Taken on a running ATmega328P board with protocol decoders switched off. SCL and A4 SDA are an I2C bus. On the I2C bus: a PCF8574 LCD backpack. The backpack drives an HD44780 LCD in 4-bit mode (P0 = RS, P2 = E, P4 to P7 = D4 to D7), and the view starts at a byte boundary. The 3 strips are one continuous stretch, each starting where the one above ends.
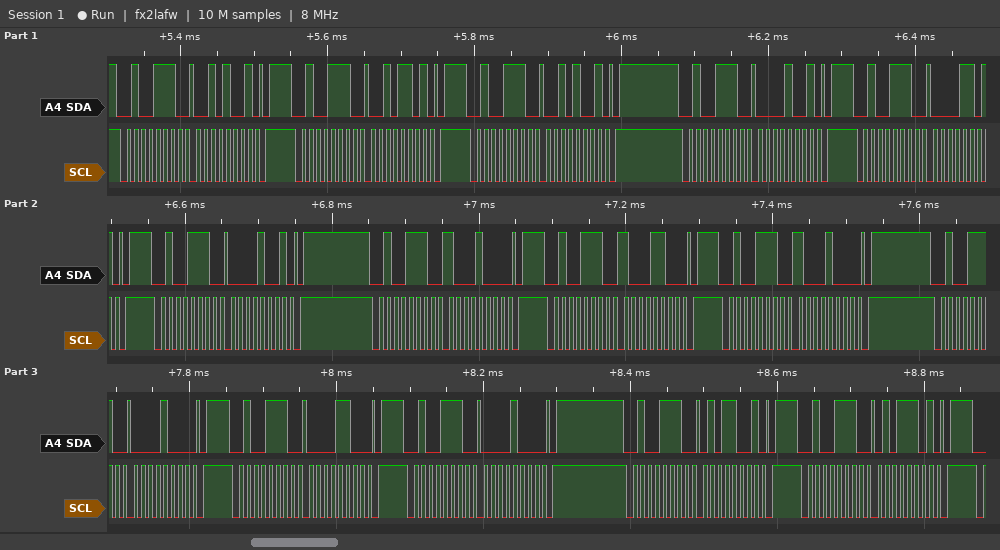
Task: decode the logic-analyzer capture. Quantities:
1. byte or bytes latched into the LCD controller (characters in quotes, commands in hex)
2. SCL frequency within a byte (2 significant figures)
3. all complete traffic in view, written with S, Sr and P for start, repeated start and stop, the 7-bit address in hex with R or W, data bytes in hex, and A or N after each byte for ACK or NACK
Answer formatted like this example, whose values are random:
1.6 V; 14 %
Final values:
' ' 0x80; 100 kHz; S 27W A 29 A P S 27W A 2D A P S 27W A 29 A P S 27W A 09 A P S 27W A 0D A P S 27W A 09 A P S 27W A 88 A P S 27W A 8C A P S 27W A 88 A P S 27W A 08 A P S 27W A 0C A P S 27W A 08 A P S 27W A 59 A P S 27W A 5D A P
